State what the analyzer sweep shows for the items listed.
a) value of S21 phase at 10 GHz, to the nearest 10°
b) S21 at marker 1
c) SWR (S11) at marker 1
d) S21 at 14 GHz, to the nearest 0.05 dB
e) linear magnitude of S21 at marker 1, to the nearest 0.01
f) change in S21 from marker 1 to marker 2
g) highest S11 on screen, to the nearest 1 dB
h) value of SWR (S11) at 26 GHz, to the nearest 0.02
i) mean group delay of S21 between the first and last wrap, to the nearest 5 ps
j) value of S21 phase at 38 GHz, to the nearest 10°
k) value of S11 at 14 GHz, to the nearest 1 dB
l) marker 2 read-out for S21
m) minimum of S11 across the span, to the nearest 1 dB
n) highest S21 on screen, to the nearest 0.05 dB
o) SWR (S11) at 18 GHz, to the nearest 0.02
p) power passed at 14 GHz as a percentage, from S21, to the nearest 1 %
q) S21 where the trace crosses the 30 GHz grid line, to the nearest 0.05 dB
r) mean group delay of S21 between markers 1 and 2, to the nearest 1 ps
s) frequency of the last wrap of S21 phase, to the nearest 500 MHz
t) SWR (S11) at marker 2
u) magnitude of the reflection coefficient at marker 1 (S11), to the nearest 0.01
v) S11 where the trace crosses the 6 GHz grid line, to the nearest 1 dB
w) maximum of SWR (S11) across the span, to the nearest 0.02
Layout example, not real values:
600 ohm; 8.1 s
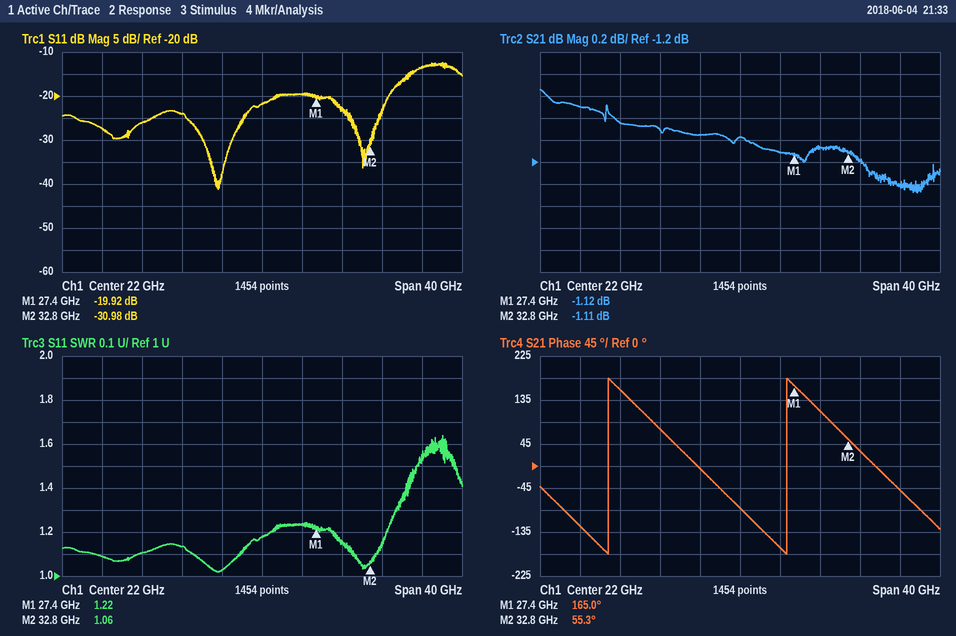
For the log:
160°; -1.12 dB; 1.22; -0.90 dB; 0.88; 0.01 dB; -12 dB; 1.24; 55 ps; -50°; -24 dB; -1.11 dB; -41 dB; -0.55 dB; 1.02; 81 %; -1.05 dB; 56 ps; 26.5 GHz; 1.06; 0.10; -27 dB; 1.64
